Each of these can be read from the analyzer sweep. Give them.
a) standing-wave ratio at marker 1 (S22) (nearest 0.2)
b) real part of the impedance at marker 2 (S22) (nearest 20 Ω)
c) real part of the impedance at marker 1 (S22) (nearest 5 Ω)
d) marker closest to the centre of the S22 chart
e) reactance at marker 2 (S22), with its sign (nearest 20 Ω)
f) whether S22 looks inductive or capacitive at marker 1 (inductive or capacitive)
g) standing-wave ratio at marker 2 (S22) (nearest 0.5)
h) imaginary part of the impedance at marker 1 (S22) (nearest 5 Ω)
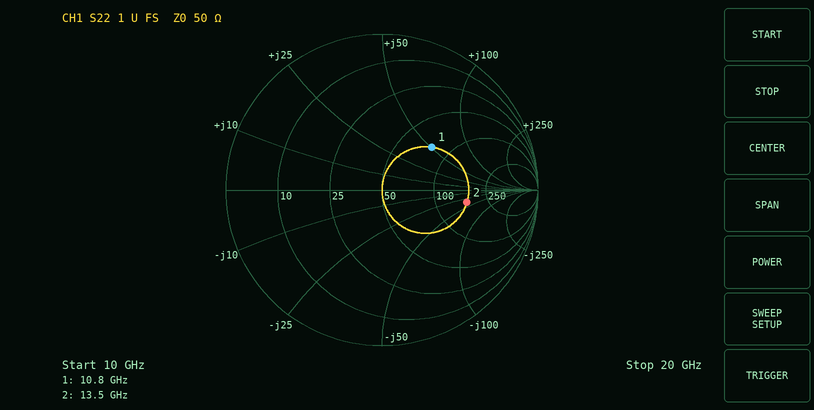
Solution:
2.4
160 Ω
75 Ω
marker 1
-40 Ω
inductive
3.5
+50 Ω
